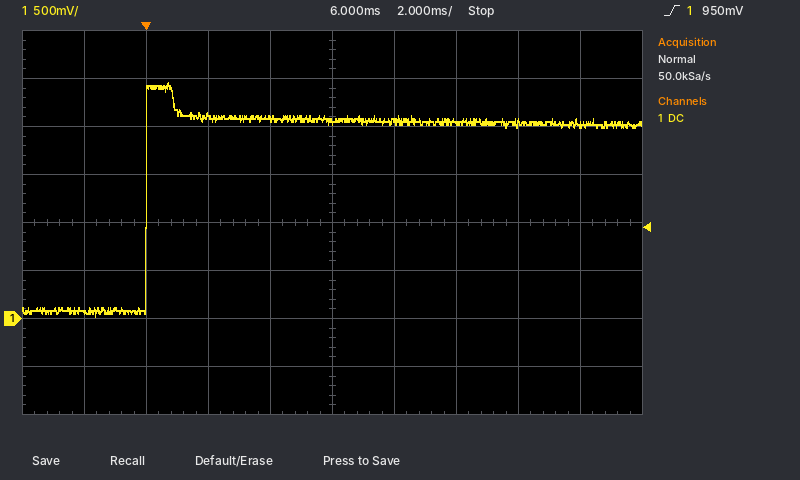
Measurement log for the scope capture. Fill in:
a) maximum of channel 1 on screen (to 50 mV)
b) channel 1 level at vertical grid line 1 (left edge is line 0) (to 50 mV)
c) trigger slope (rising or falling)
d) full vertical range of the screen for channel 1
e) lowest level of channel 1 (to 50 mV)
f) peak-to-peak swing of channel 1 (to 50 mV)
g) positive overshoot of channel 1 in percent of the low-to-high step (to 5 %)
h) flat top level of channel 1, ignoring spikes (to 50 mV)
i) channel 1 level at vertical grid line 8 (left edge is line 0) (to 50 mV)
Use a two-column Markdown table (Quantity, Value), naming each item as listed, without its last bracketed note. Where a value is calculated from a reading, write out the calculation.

| Quantity | Value |
|---|---|
| maximum of channel 1 on screen | 2.45 V |
| channel 1 level at vertical grid line 1 (left edge is line 0) | 50 mV |
| trigger slope | rising |
| full vertical range of the screen for channel 1 | 4 V |
| lowest level of channel 1 | 0 mV |
| peak-to-peak swing of channel 1 | 2.45 V − (0 mV) = 2.45 V |
| positive overshoot of channel 1 in percent of the low-to-high step | 20 % |
| flat top level of channel 1, ignoring spikes | 2.05 V |
| channel 1 level at vertical grid line 8 (left edge is line 0) | 2.05 V |
